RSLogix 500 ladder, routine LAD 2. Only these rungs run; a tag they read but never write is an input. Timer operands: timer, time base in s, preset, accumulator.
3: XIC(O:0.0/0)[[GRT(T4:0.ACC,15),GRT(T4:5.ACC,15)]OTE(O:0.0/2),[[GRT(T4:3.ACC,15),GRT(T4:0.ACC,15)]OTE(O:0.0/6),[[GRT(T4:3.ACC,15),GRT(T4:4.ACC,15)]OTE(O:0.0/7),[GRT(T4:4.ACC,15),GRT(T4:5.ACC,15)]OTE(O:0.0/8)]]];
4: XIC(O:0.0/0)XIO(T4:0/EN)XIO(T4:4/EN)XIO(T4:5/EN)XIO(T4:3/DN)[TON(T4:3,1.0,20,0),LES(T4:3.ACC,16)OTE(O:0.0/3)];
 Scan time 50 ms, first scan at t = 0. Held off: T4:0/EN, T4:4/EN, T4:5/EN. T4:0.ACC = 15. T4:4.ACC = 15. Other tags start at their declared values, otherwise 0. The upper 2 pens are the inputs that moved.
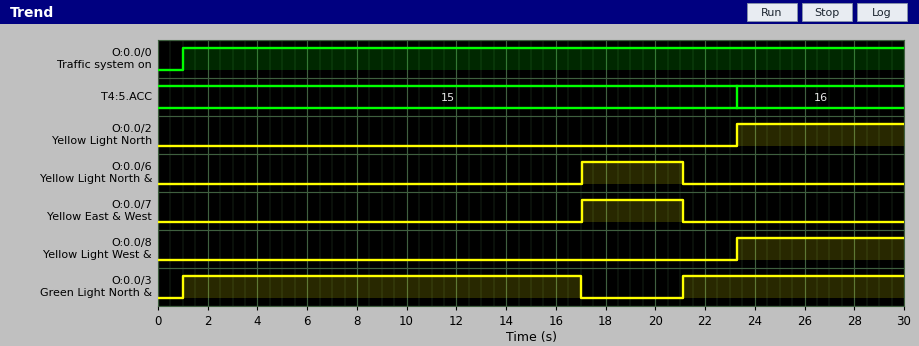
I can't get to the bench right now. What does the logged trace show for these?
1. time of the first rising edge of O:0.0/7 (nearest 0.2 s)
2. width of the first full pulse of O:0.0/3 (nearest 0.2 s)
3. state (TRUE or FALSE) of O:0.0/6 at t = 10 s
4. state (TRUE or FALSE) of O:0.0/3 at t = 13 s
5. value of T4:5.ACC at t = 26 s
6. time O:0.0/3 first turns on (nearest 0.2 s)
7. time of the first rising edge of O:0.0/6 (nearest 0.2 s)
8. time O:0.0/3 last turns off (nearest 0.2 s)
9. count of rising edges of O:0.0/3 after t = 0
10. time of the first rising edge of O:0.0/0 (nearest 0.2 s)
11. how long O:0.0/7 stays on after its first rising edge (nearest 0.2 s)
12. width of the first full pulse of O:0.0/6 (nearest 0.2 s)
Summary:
17.0 s
16.0 s
FALSE
TRUE
16
1.0 s
17.0 s
17.0 s
2
1.0 s
4.0 s
4.0 s
